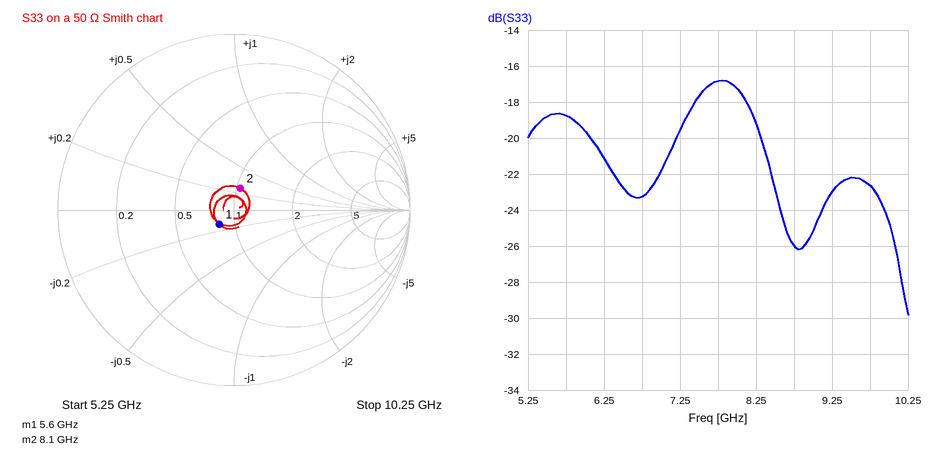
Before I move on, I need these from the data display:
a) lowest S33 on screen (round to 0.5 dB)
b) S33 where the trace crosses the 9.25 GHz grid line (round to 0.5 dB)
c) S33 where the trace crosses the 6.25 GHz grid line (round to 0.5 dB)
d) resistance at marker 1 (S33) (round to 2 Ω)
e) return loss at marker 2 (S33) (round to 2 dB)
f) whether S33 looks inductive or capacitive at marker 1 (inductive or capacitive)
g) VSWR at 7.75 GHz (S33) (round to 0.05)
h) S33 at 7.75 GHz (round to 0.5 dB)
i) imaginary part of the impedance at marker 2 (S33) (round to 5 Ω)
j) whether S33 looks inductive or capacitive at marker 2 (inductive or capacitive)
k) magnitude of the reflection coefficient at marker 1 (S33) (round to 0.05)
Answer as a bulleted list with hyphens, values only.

- -30.0 dB
- -23.0 dB
- -21.0 dB
- 42 Ω
- 18 dB
- capacitive
- 1.35
- -17.0 dB
- +15 Ω
- inductive
- 0.10
